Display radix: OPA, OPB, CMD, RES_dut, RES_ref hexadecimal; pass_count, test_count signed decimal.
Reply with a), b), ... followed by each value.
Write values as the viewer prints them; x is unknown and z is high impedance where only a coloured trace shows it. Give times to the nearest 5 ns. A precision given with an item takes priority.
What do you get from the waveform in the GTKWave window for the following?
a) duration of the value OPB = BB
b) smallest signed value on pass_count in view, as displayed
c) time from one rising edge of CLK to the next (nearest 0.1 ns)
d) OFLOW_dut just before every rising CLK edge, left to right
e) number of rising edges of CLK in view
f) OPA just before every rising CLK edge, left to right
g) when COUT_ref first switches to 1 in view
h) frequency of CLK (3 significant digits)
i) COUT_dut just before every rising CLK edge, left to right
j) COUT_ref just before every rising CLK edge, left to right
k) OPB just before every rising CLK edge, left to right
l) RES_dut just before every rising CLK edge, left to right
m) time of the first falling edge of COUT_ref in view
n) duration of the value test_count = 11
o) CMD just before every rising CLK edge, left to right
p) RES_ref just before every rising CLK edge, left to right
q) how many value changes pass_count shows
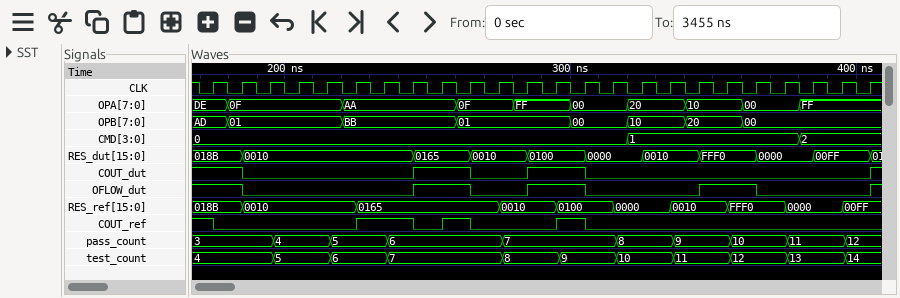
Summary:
a) 40 ns
b) 3
c) 10 ns
d) 1 1 0 0 0 0 0 0 1 1 0 0 1 1 0 0 0 0 1 1 0 0 0 0
e) 24
f) DE, 0F, 0F, 0F, 0F, AA, AA, AA, AA, 0F, 0F, FF, FF, 00, 00, 20, 20, 10, 10, 00, 00, FF, FF, FF
g) 225 ns
h) 100 MHz
i) 1 1 0 0 0 0 0 0 1 1 0 0 1 1 0 0 0 0 0 0 0 0 0 0
j) 1 0 0 0 0 0 1 1 0 1 0 0 0 1 0 0 0 0 0 0 0 0 0 0
k) AD, 01, 01, 01, 01, BB, BB, BB, BB, 01, 01, 01, 01, 00, 00, 10, 10, 20, 20, 00, 00, 00, 00, 00
l) 018B, 018B, 0010, 0010, 0010, 0010, 0010, 0010, 0165, 0165, 0010, 0010, 0100, 0100, 0000, 0000, 0010, 0010, FFF0, FFF0, 0000, 0000, 00FF, 00FF
m) 175 ns
n) 20 ns
o) 0, 0, 0, 0, 0, 0, 0, 0, 0, 0, 0, 0, 0, 0, 0, 1, 1, 1, 1, 1, 1, 2, 2, 2
p) 018B, 018B, 0010, 0010, 0010, 0010, 0165, 0165, 0165, 0165, 0165, 0010, 0010, 0100, 0100, 0000, 0000, 0010, 0010, FFF0, FFF0, 0000, 0000, 00FF
q) 9
